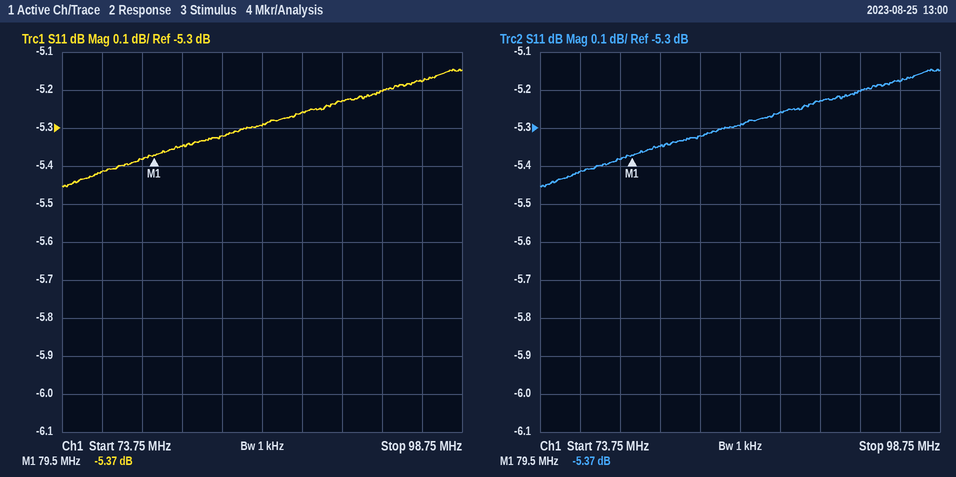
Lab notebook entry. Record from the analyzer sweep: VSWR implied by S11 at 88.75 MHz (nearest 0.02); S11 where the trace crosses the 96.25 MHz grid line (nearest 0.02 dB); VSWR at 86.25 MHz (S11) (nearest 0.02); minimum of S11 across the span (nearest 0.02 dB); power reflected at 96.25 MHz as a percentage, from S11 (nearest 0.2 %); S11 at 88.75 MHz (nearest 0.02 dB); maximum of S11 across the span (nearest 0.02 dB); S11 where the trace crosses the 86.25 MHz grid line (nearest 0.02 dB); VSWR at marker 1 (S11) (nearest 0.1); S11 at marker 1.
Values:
3.40
-5.18 dB
3.38
-5.46 dB
30.4 %
-5.26 dB
-5.14 dB
-5.30 dB
3.3
-5.37 dB
